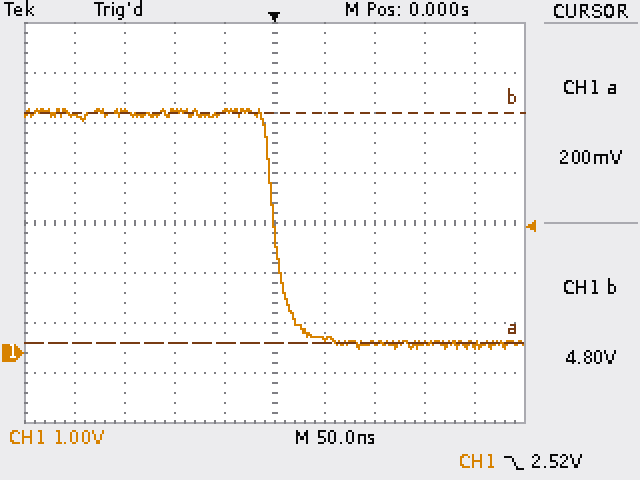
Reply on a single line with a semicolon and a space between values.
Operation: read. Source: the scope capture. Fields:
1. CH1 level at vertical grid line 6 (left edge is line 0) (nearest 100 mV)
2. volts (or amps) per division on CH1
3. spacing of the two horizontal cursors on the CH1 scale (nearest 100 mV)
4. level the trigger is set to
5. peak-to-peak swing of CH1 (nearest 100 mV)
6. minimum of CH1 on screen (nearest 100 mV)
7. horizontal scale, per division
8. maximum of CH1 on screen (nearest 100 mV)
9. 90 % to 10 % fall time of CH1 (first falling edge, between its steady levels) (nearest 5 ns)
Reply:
300 mV; 1 V; 4.6 V; 2.52 V; 4.8 V; 100 mV; 50 ns; 4.9 V; 30 ns
